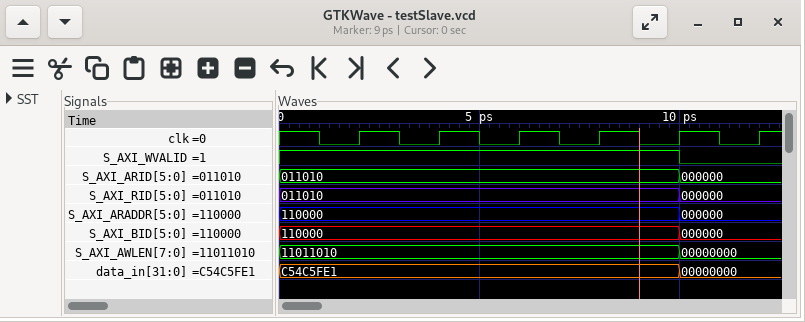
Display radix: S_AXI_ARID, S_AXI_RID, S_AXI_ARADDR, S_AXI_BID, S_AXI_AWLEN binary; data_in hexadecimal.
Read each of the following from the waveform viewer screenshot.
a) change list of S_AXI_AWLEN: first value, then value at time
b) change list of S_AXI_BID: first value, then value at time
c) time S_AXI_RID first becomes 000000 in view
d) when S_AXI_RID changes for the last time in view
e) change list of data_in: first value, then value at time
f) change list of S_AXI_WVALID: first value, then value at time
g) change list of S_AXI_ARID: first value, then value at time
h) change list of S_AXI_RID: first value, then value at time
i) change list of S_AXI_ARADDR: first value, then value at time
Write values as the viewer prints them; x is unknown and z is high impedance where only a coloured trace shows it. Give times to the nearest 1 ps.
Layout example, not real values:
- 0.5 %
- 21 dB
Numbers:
- 11011010, 00000000 at 10 ps
- 110000, 000000 at 10 ps
- 10 ps
- 10 ps
- C54C5FE1, 00000000 at 10 ps
- 1, 0 at 10 ps
- 011010, 000000 at 10 ps
- 011010, 000000 at 10 ps
- 110000, 000000 at 10 ps
